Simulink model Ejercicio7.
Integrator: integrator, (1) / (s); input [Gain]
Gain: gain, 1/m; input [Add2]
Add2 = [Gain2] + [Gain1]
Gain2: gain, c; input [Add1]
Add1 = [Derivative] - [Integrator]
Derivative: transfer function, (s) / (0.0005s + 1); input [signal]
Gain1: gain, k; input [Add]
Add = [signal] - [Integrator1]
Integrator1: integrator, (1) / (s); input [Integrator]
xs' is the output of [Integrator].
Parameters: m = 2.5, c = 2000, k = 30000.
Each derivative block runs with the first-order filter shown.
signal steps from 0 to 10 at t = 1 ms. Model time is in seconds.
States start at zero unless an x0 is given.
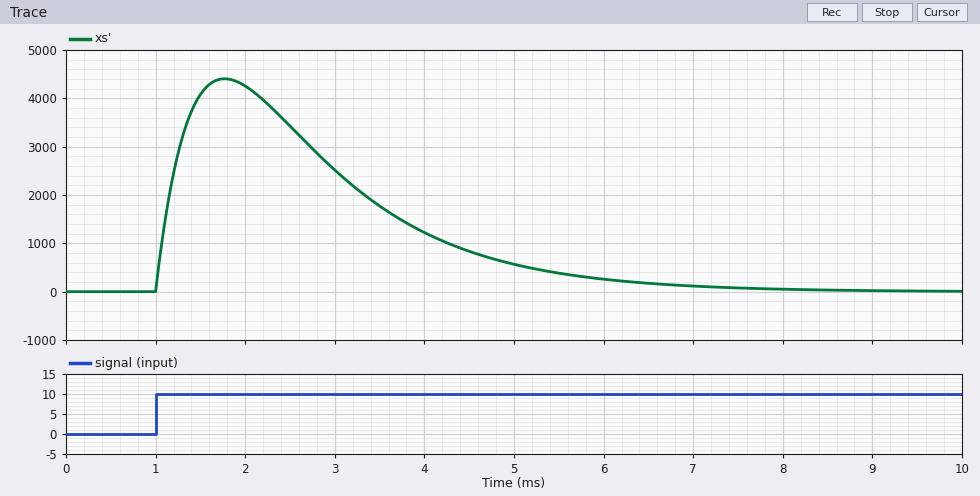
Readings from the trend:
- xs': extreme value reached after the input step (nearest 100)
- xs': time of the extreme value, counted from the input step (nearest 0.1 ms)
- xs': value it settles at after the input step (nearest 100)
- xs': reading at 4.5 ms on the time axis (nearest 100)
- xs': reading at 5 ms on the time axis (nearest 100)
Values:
4400
0.8 ms
0
800
600
